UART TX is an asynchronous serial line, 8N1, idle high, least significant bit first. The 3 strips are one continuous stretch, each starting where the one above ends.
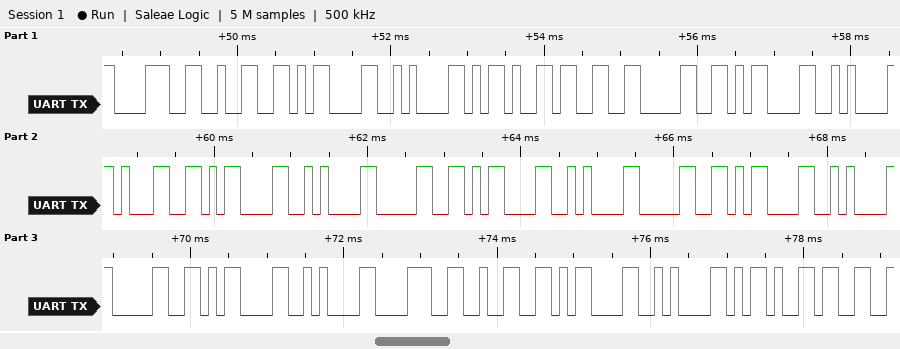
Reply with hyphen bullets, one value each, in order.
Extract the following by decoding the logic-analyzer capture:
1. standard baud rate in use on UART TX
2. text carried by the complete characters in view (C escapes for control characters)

- 9600 baud
- "82\r\n-30\r\n1\r\n0\r\n0\r\n0\r\n82\r\n-3"
